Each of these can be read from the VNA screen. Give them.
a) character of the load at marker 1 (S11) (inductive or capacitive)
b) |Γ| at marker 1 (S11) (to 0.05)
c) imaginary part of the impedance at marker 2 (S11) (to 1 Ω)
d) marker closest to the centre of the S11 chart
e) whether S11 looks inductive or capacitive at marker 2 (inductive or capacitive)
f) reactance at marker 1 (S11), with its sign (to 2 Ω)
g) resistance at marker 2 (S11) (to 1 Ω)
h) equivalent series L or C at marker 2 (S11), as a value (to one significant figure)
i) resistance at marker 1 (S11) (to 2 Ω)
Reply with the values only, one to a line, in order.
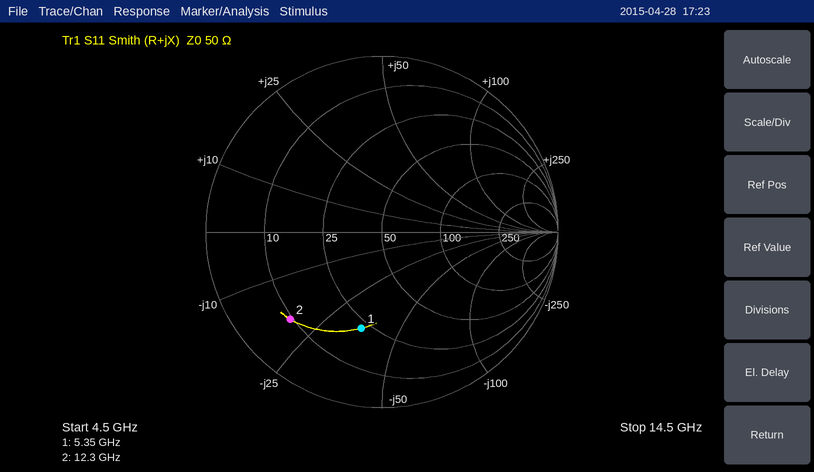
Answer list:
capacitive
0.55
-19 Ω
marker 1
capacitive
-36 Ω
9 Ω
700 fF
22 Ω
